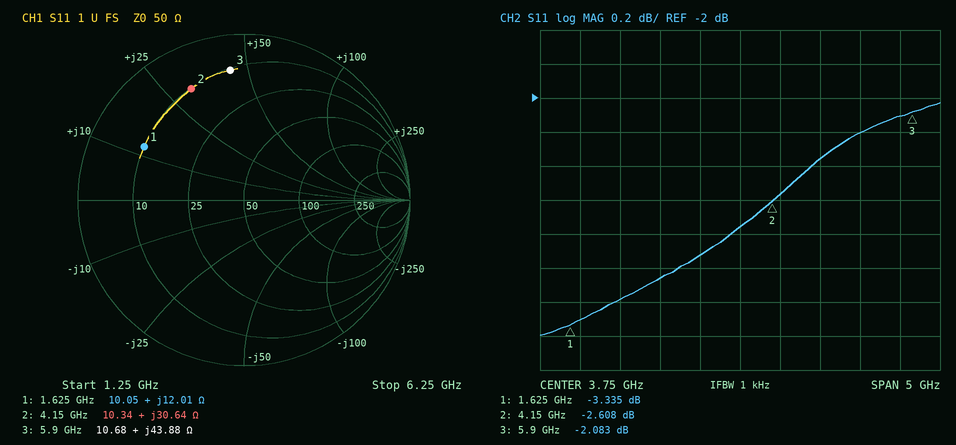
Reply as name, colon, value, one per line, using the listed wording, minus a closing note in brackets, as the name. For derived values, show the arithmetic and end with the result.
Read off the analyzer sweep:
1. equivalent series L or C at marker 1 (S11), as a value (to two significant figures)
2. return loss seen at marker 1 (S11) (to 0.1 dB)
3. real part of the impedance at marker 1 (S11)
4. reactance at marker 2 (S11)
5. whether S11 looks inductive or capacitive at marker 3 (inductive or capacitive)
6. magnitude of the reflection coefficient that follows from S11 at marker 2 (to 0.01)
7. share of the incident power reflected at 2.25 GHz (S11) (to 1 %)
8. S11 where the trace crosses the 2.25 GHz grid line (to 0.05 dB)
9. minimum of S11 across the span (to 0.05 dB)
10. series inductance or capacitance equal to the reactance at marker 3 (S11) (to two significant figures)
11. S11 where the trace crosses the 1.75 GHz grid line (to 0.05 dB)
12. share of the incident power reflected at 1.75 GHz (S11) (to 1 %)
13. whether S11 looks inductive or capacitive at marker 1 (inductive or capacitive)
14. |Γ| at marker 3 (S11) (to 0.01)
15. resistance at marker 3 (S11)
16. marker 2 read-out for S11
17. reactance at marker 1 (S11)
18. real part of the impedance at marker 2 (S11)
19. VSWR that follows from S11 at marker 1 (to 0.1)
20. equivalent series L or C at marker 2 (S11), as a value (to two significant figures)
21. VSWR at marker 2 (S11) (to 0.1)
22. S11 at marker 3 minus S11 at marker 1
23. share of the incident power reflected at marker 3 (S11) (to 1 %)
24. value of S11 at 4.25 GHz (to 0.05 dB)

equivalent series L or C at marker 1 (S11), as a value: L = 12.01 Ω/(2π × 1.625 GHz) ≈ 1.2 nH
return loss seen at marker 1 (S11): 3.3 dB
real part of the impedance at marker 1: 10.05 Ω
reactance at marker 2: +30.64 Ω
whether S11 looks inductive or capacitive at marker 3: inductive
magnitude of the reflection coefficient that follows from S11 at marker 2: 10^(-2.608/20) ≈ 0.74
share of the incident power reflected at 2.25 GHz (S11): 10^(-3.2/10) ≈ 48 %
S11 where the trace crosses the 2.25 GHz grid line: -3.20 dB
minimum of S11 across the span: -3.40 dB
series inductance or capacitance equal to the reactance at marker 3 (S11): L = 43.88 Ω/(2π × 5.9 GHz) ≈ 1.2 nH
S11 where the trace crosses the 1.75 GHz grid line: -3.30 dB
share of the incident power reflected at 1.75 GHz (S11): 10^(-3.3/10) ≈ 47 %
whether S11 looks inductive or capacitive at marker 1: inductive
|Γ| at marker 3 (S11): 0.79
resistance at marker 3: 10.68 Ω
marker 2 read-out for S11: -2.608 dB
reactance at marker 1: +12.01 Ω
real part of the impedance at marker 2: 10.34 Ω
VSWR that follows from S11 at marker 1: (1 + 0.6812)/(1 − 0.6812) ≈ 5.3
equivalent series L or C at marker 2 (S11), as a value: L = 30.64 Ω/(2π × 4.15 GHz) ≈ 1.2 nH
VSWR at marker 2 (S11): 6.7
S11 at marker 3 minus S11 at marker 1: -2.083 − (-3.335) = 1.252 dB
share of the incident power reflected at marker 3 (S11): 10^(-2.083/10) ≈ 62 %
value of S11 at 4.25 GHz: -2.55 dB
